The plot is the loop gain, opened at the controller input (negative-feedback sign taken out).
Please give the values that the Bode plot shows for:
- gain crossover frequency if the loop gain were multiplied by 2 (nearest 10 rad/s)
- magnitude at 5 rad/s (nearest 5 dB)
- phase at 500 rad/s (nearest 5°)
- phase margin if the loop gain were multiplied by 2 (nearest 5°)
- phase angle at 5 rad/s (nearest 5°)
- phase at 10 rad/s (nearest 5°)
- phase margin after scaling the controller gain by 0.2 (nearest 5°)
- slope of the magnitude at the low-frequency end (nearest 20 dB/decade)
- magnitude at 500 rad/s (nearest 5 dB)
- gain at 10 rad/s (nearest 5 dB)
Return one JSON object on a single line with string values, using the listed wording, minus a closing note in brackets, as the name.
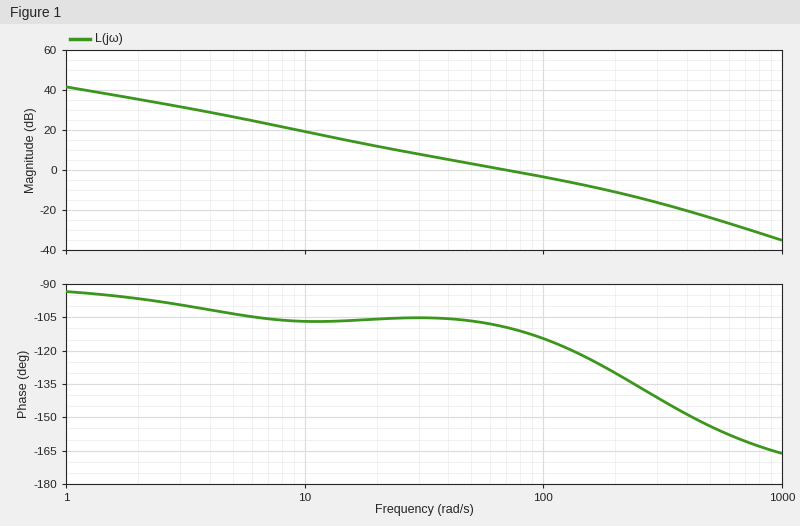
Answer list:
{"gain crossover frequency if the loop gain were multiplied by 2": "130 rad/s", "magnitude at 5 rad/s": "25 dB", "phase at 500 rad/s": "-155°", "phase margin if the loop gain were multiplied by 2": "60°", "phase angle at 5 rad/s": "-105°", "phase at 10 rad/s": "-105°", "phase margin after scaling the controller gain by 0.2": "75°", "slope of the magnitude at the low-frequency end": "-20 dB/decade", "magnitude at 500 rad/s": "-25 dB", "gain at 10 rad/s": "20 dB"}
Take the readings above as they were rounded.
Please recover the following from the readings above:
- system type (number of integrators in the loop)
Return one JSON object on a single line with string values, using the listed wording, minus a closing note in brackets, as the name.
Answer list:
{"system type": "1"}
